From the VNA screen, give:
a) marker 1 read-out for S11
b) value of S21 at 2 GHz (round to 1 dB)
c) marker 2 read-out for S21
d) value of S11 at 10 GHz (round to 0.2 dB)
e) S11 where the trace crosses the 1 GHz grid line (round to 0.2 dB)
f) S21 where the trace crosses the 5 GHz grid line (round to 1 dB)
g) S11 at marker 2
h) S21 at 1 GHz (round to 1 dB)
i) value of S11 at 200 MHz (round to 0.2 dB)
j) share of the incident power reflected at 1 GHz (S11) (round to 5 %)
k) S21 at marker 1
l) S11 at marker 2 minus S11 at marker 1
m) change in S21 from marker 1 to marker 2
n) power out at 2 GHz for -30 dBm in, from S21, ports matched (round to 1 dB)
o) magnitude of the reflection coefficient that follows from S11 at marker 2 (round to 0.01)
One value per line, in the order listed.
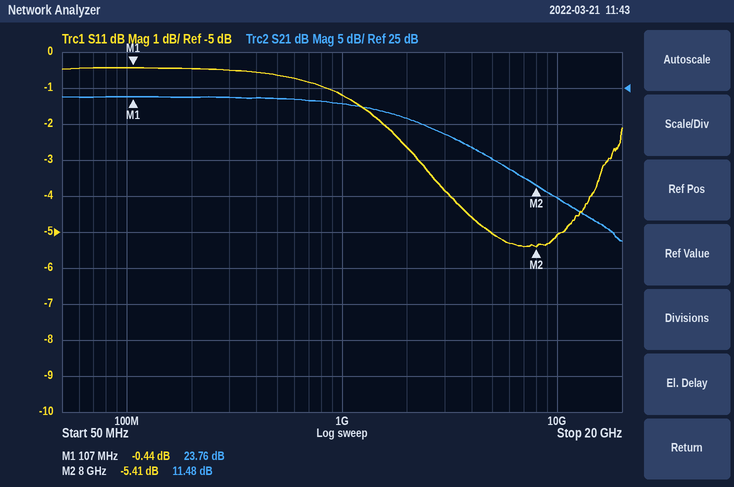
-0.44 dB
21 dB
11.48 dB
-5.0 dB
-1.2 dB
15 dB
-5.41 dB
23 dB
-0.4 dB
75 %
23.76 dB
-4.97 dB
-12.28 dB
-9 dBm
0.54
